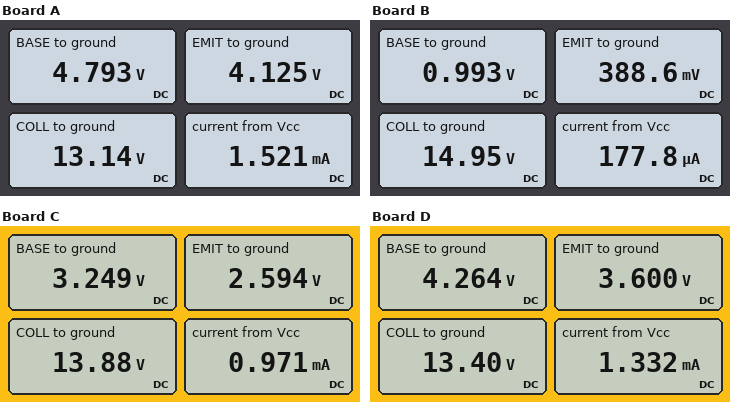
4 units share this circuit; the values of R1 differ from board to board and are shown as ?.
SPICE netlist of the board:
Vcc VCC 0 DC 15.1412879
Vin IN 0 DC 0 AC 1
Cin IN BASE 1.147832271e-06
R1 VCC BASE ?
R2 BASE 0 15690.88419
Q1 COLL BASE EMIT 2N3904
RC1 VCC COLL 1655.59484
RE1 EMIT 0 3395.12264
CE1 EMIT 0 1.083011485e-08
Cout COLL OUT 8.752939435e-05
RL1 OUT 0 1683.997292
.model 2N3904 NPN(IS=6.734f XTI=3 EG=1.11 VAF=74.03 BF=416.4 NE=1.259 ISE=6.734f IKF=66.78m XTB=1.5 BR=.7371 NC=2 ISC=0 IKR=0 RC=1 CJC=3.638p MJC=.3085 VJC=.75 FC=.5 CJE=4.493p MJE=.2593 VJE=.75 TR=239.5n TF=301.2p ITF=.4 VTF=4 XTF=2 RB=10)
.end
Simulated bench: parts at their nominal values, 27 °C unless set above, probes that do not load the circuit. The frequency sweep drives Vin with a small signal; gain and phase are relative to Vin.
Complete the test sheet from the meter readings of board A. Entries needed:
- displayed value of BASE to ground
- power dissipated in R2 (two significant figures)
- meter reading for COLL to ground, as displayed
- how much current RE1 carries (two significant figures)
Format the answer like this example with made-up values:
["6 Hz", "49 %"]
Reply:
["4.793 V", "1.5 mW", "13.14 V", "1.2 mA"]
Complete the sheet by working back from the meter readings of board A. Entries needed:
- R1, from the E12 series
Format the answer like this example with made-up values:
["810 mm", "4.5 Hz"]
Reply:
["33 kΩ"]
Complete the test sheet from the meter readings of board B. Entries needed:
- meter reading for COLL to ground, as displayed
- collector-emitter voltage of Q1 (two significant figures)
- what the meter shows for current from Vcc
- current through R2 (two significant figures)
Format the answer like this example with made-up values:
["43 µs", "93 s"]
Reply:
["14.95 V", "15 V", "177.8 µA", "63 µA"]
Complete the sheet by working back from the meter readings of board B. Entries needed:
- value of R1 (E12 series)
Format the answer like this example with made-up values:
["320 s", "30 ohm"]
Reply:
["220 kΩ"]
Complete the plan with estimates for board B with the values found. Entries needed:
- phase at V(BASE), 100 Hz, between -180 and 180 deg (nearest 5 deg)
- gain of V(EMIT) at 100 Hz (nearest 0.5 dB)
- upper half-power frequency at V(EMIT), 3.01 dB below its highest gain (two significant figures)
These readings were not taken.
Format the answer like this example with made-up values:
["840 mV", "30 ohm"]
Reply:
["5 deg", "-0.5 dB", "69 kHz"]
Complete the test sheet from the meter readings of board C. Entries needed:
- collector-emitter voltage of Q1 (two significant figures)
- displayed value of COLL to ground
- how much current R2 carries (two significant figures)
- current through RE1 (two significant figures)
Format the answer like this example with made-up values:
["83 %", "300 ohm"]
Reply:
["11 V", "13.88 V", "210 µA", "760 µA"]
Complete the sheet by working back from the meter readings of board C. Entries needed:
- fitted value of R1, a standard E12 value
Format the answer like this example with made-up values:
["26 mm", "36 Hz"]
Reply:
["56 kΩ"]
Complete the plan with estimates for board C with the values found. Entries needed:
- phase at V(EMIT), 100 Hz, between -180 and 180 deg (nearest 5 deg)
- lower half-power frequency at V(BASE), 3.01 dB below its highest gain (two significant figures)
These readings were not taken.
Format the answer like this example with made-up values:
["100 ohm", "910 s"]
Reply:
["5 deg", "12 Hz"]
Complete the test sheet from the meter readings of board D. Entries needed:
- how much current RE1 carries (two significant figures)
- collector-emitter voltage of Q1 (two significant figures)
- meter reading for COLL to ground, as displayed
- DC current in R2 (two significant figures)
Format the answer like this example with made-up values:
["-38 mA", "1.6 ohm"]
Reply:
["1.1 mA", "9.8 V", "13.40 V", "270 µA"]
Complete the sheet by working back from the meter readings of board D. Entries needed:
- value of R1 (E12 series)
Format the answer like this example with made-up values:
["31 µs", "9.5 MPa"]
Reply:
["39 kΩ"]
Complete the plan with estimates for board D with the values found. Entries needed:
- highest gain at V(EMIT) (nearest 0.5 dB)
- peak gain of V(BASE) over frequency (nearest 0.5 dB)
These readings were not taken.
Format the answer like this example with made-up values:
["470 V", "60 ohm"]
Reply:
["0 dB", "0 dB"]
